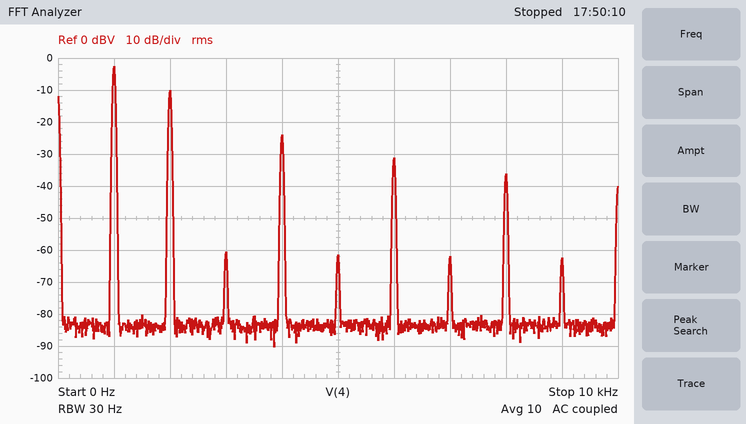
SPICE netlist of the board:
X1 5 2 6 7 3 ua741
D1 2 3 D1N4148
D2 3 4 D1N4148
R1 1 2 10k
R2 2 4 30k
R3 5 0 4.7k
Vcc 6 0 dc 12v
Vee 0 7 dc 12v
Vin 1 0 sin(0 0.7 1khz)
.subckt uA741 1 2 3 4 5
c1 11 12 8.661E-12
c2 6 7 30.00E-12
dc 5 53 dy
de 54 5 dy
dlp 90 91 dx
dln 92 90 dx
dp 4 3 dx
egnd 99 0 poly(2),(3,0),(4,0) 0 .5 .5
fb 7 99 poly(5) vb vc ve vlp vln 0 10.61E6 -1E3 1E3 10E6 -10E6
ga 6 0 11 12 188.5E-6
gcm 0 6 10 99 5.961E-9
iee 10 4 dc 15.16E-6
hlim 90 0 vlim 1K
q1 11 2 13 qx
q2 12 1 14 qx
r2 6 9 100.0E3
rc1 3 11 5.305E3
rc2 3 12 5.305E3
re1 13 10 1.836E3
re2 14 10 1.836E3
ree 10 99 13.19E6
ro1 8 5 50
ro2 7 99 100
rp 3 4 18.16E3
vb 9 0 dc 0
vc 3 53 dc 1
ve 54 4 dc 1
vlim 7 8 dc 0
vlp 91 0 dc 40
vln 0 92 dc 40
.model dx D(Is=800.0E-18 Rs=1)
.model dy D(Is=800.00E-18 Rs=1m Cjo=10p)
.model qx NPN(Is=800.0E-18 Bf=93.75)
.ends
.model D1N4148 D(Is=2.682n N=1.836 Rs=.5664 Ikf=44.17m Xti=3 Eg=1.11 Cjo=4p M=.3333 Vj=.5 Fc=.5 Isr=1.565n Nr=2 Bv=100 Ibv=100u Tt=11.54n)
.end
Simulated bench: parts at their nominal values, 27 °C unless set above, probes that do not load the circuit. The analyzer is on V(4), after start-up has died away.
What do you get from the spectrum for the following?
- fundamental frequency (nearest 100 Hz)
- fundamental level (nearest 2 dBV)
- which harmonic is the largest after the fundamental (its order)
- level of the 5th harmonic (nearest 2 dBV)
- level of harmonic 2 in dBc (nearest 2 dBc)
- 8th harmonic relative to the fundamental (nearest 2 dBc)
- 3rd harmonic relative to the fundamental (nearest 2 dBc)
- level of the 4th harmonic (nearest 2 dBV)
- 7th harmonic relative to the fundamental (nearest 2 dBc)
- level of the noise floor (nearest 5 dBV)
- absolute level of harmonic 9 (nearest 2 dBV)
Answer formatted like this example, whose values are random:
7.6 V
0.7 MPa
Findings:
1.0 kHz
-2 dBV
2
-62 dBV
-8 dBc
-34 dBc
-58 dBc
-24 dBV
-60 dBc
-85 dBV
-62 dBV
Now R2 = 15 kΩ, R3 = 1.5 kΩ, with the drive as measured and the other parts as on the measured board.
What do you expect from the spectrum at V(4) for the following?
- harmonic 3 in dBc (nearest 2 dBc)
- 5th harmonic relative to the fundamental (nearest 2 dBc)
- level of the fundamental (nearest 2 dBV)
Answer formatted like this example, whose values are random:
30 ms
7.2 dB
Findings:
-56 dBc
-56 dBc
-8 dBV
